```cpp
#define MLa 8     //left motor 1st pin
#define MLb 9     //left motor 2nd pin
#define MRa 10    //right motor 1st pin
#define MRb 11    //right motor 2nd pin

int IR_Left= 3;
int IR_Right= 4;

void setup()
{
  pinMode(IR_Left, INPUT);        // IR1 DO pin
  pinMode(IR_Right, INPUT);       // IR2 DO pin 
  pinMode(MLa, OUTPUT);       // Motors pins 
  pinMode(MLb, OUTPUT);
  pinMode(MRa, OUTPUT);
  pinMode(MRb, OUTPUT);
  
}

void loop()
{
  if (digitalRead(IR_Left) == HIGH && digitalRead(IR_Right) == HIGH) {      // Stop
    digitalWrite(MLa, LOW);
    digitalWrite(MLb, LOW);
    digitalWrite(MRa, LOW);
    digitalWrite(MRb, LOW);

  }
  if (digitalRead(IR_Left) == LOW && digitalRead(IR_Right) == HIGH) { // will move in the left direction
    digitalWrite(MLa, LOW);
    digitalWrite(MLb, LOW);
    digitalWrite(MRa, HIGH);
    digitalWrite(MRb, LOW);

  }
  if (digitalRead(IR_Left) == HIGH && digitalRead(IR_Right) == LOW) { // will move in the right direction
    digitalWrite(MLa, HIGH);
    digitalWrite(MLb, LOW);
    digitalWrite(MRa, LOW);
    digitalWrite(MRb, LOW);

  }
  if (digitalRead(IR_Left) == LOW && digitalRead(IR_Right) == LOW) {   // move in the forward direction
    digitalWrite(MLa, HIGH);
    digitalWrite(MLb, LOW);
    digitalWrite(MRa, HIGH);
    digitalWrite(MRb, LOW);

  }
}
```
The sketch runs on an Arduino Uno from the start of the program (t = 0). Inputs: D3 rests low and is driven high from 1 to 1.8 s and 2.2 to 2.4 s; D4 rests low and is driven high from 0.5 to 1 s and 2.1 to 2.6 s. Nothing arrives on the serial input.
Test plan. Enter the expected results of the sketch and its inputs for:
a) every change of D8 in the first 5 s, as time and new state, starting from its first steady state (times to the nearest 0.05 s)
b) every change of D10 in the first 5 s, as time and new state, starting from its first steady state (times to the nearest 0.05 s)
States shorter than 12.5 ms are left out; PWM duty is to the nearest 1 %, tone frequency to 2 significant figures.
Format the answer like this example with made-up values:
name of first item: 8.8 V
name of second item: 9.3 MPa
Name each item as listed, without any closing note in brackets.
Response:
every change of D8 in the first 5 s, as time and new state, starting from its first steady state: 0 s high; 0.5 s low; 1 s high; 2.1 s low; 2.6 s high
every change of D10 in the first 5 s, as time and new state, starting from its first steady state: 0 s high; 1 s low; 1.8 s high; 2.2 s low; 2.4 s high
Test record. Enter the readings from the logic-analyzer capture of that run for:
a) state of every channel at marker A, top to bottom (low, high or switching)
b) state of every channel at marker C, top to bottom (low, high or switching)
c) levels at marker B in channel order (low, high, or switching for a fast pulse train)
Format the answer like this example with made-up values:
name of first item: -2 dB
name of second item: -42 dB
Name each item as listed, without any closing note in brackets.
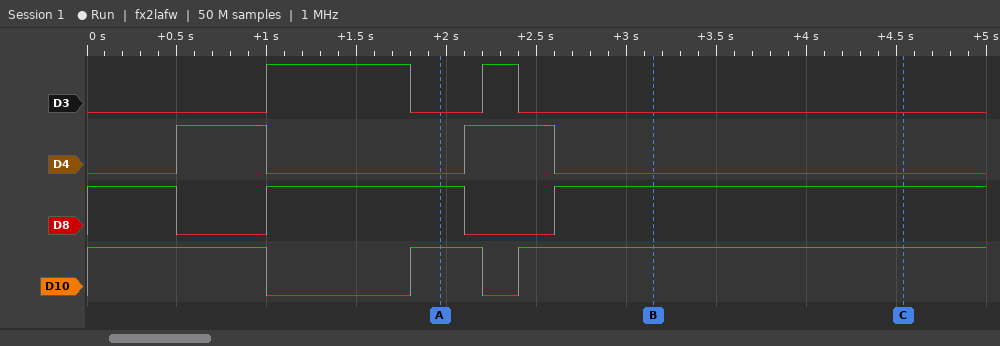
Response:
state of every channel at marker A, top to bottom: D3 low, D4 low, D8 high, D10 high
state of every channel at marker C, top to bottom: D3 low, D4 low, D8 high, D10 high
levels at marker B in channel order: D3 low, D4 low, D8 high, D10 high
